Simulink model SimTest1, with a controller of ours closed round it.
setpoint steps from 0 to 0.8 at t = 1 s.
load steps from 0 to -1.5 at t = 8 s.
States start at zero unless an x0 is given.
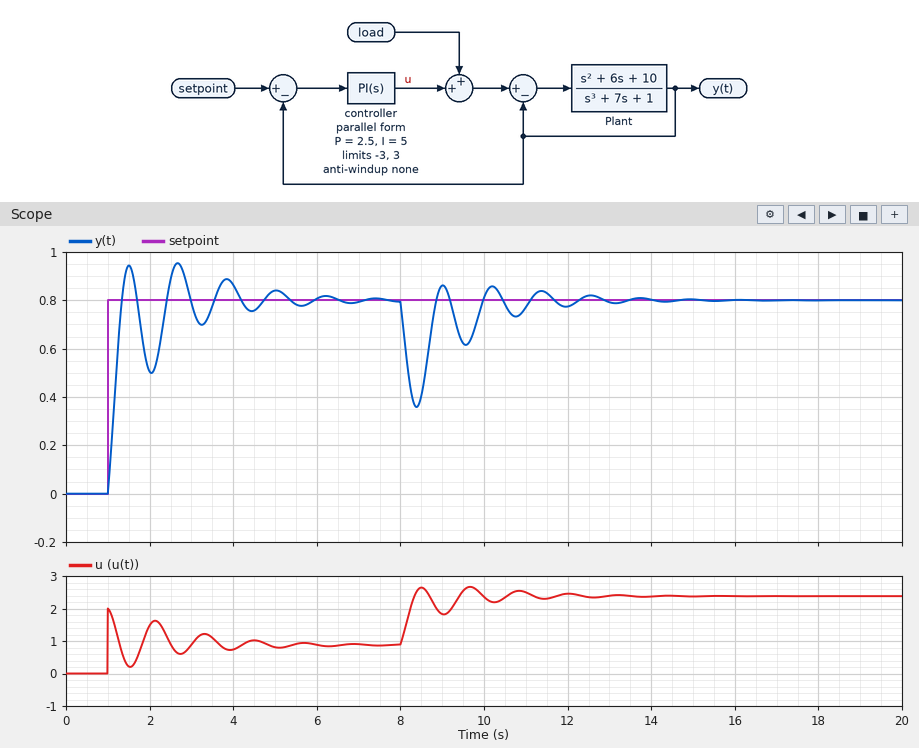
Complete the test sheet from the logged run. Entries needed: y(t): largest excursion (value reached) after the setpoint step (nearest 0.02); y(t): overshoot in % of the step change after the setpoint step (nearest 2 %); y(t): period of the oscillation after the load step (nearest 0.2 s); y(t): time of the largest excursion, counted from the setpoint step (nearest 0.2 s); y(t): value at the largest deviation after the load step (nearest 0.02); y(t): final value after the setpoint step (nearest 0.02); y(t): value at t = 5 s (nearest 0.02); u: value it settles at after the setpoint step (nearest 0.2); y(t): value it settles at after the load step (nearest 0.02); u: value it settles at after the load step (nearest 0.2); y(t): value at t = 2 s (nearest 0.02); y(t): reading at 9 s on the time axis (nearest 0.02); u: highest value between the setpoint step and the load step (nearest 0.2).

0.96
20 %
1.2 s
1.6 s
0.36
0.80
0.84
0.8
0.80
2.4
0.50
0.86
2.0
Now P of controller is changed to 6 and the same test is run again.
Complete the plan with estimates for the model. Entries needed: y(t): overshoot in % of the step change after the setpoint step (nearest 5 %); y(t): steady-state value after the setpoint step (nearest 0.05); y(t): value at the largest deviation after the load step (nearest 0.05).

15 %
0.80
0.55
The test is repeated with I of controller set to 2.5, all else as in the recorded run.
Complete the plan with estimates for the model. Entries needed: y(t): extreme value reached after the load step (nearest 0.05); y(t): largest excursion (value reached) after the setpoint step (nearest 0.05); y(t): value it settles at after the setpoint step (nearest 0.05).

0.30
0.85
0.80
